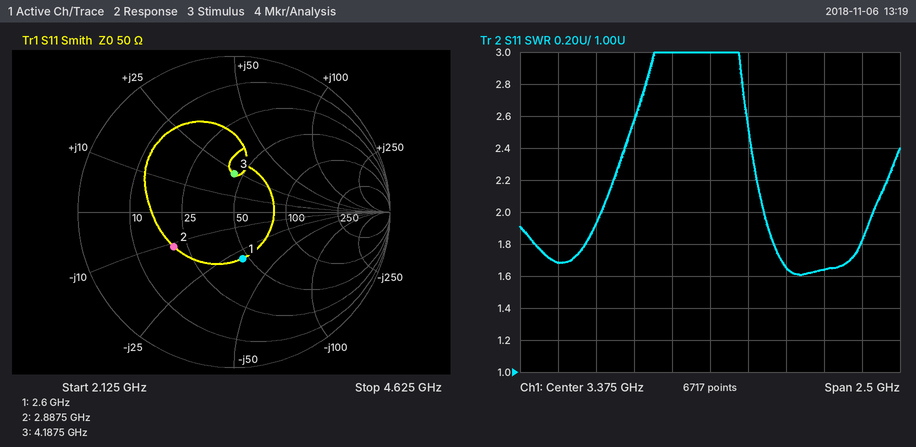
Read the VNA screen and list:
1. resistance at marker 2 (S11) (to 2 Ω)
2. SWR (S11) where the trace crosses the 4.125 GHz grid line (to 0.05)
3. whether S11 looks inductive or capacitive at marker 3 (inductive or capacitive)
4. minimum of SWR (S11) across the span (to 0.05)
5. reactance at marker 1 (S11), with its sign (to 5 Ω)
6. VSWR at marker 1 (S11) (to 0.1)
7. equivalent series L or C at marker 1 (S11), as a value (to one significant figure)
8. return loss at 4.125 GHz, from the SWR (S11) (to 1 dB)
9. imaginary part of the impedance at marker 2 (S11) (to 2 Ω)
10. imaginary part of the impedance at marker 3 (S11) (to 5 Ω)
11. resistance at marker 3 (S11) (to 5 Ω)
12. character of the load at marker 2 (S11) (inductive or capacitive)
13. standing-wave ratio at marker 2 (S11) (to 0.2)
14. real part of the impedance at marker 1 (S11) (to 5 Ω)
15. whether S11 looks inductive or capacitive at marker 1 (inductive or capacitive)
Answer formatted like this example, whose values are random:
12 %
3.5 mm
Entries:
20 Ω
1.65
inductive
1.60
-30 Ω
1.9
2 pF
12 dB
-12 Ω
+25 Ω
45 Ω
capacitive
2.6
45 Ω
capacitive
